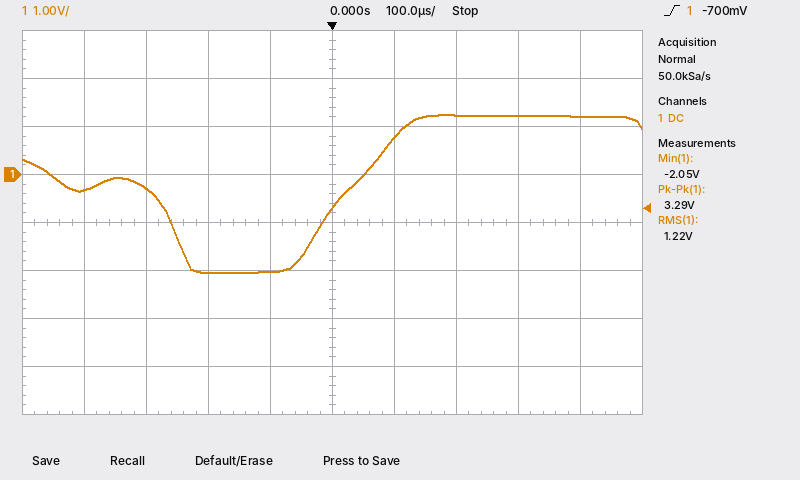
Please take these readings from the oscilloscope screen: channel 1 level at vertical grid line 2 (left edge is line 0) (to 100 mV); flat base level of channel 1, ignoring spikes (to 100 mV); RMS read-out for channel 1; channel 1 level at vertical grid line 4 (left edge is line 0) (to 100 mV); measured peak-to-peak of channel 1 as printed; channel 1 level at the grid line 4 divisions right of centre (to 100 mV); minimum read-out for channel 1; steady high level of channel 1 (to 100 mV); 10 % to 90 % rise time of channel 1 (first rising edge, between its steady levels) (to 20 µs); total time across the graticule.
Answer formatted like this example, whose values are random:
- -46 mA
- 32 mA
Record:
- -300 mV
- -2.0 V
- 1.22 V
- -2.0 V
- 3.29 V
- 1.2 V
- -2.05 V
- 1.2 V
- 160 µs
- 1 ms
